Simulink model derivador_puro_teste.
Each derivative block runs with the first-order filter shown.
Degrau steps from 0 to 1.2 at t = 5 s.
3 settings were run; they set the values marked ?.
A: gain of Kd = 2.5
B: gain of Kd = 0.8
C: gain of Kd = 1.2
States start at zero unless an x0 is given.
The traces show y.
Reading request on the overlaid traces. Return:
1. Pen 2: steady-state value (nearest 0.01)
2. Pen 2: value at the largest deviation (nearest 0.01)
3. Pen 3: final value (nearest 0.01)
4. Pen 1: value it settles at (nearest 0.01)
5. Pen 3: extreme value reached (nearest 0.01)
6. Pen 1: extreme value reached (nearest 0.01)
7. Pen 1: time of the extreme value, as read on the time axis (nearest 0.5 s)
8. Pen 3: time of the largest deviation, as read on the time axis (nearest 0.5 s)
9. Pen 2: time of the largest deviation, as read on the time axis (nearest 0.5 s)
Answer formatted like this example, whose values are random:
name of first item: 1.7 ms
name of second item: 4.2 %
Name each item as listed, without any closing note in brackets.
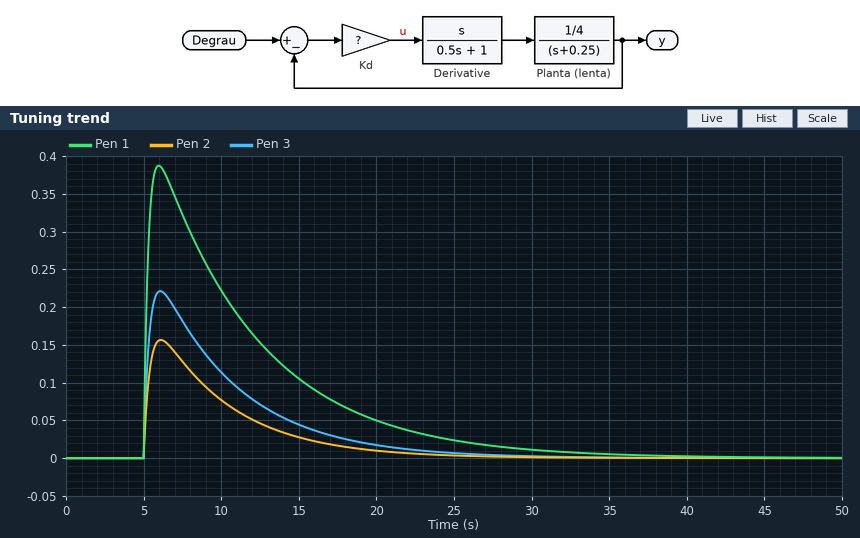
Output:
Pen 2: steady-state value: 0.00
Pen 2: value at the largest deviation: 0.16
Pen 3: final value: 0.00
Pen 1: value it settles at: 0.00
Pen 3: extreme value reached: 0.22
Pen 1: extreme value reached: 0.39
Pen 1: time of the extreme value, as read on the time axis: 6.0 s
Pen 3: time of the largest deviation, as read on the time axis: 6.0 s
Pen 2: time of the largest deviation, as read on the time axis: 6.0 s
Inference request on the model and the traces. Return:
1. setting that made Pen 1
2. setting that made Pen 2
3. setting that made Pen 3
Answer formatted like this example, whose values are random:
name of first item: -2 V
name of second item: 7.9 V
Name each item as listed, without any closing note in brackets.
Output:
setting that made Pen 1: A
setting that made Pen 2: B
setting that made Pen 3: C
